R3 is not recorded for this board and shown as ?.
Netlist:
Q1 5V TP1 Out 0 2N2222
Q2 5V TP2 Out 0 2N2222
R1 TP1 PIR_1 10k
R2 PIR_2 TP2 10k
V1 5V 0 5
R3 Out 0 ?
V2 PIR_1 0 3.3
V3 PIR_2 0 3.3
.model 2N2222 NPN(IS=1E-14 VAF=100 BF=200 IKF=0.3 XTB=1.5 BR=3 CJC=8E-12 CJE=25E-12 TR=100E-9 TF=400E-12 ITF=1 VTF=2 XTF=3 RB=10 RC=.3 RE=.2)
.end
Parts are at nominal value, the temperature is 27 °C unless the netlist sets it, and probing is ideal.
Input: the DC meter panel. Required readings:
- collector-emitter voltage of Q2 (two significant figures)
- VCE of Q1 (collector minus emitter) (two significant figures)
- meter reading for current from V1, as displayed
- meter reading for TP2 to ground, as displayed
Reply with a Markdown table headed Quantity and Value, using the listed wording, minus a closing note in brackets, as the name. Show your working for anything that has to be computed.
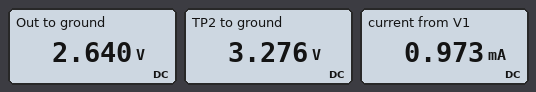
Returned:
| Quantity | Value |
|---|---|
| collector-emitter voltage of Q2 | 5 V - 2.64 V = 2.4 V |
| VCE of Q1 (collector minus emitter) | 5 V - 2.64 V = 2.4 V |
| meter reading for current from V1, as displayed | 0.973 mA |
| meter reading for TP2 to ground, as displayed | 3.276 V |
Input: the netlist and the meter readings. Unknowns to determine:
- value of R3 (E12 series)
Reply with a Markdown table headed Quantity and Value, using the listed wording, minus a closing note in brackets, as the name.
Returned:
| Quantity | Value |
|---|---|
| value of R3 | 2.7 kΩ |
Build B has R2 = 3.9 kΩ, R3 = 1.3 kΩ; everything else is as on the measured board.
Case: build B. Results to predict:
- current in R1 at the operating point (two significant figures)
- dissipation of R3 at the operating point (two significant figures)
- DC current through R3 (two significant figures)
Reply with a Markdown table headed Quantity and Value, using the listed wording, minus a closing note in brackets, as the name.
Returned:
| Quantity | Value |
|---|---|
| current in R1 at the operating point | 3.7 µA |
| dissipation of R3 at the operating point | 5.3 mW |
| DC current through R3 | 2.0 mA |
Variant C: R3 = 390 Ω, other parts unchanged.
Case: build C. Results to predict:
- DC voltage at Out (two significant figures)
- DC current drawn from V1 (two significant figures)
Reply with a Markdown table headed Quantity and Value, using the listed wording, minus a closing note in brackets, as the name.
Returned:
| Quantity | Value |
|---|---|
| DC voltage at Out | 2.5 V |
| DC current drawn from V1 | 6.3 mA |
